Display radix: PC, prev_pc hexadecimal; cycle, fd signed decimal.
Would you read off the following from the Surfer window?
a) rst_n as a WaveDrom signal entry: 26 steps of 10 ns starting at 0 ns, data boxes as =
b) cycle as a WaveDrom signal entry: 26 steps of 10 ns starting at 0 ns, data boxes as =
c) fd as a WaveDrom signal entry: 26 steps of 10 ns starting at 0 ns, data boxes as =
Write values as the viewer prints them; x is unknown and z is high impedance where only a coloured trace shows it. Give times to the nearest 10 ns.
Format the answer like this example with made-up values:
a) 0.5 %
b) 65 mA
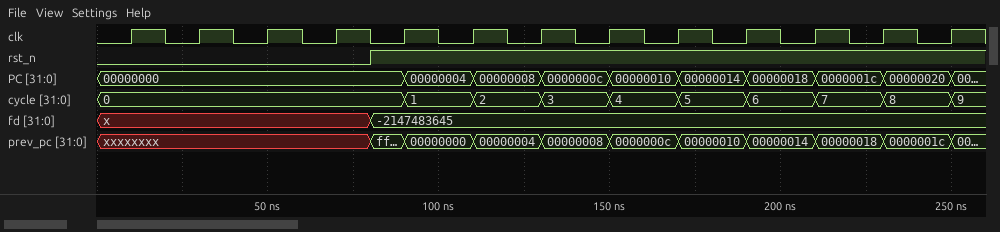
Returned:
a) {name: 'rst_n', wave: '0.......1.................'}
b) {name: 'cycle', wave: '=........=.=.=.=.=.=.=.=.=', data: '0 1 2 3 4 5 6 7 8 9'}
c) {name: 'fd', wave: 'x.......=.................', data: '-2147483645'}
